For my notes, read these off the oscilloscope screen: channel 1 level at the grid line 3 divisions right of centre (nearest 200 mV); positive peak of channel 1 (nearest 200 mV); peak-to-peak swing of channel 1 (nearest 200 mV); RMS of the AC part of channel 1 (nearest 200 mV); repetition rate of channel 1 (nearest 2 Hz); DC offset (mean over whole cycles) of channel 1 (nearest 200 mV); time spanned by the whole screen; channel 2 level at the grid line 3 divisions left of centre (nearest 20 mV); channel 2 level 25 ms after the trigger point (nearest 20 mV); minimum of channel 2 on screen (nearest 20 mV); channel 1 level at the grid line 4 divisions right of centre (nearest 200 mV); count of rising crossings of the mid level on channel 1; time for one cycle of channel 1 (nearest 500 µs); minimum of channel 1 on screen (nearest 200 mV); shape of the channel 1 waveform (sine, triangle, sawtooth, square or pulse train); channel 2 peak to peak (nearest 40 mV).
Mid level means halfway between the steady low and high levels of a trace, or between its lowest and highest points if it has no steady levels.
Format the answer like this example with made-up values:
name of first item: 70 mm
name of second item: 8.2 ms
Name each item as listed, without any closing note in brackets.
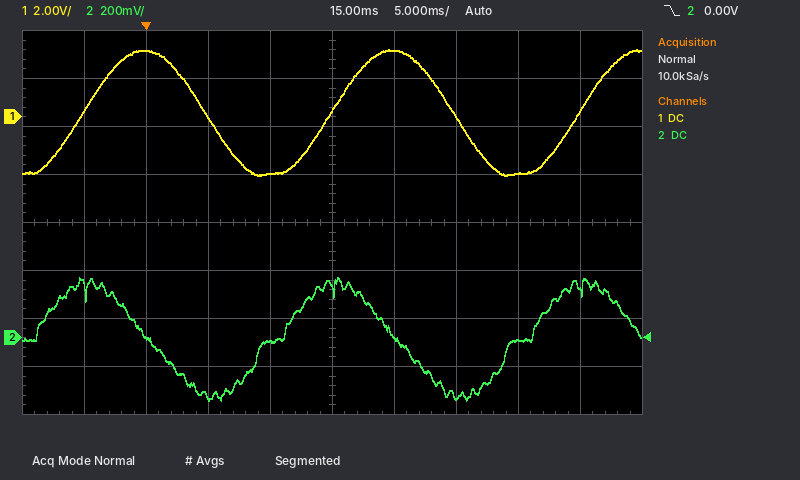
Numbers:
channel 1 level at the grid line 3 divisions right of centre: -2.4 V
positive peak of channel 1: 2.8 V
peak-to-peak swing of channel 1: 5.2 V
RMS of the AC part of channel 1: 1.8 V
repetition rate of channel 1: 50 Hz
DC offset (mean over whole cycles) of channel 1: 200 mV
time spanned by the whole screen: 50 ms
channel 2 level at the grid line 3 divisions left of centre: 0 mV
channel 2 level 25 ms after the trigger point: -240 mV
minimum of channel 2 on screen: -260 mV
channel 1 level at the grid line 4 divisions right of centre: 200 mV
count of rising crossings of the mid level on channel 1: 3
time for one cycle of channel 1: 20.0 ms
minimum of channel 1 on screen: -2.4 V
shape of the channel 1 waveform: sine
channel 2 peak to peak: 520 mV
